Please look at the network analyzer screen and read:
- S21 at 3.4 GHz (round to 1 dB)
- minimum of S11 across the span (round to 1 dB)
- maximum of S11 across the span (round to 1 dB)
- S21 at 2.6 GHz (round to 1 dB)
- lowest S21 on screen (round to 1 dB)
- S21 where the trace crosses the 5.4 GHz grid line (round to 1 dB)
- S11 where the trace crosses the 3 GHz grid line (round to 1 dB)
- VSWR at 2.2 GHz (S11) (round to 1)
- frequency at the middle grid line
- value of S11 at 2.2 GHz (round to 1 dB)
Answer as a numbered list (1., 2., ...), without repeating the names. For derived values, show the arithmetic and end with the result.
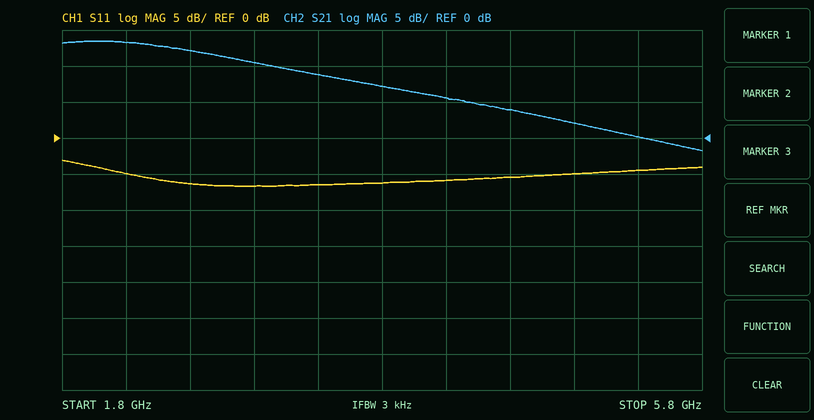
1. 9 dB
2. -7 dB
3. -3 dB
4. 12 dB
5. -2 dB
6. 0 dB
7. -7 dB
8. |Γ| = 10^(-5/20) = 0.5623; VSWR = (1 + 0.5623)/(1 − 0.5623) ≈ 4
9. 3.8 GHz
10. -5 dB
